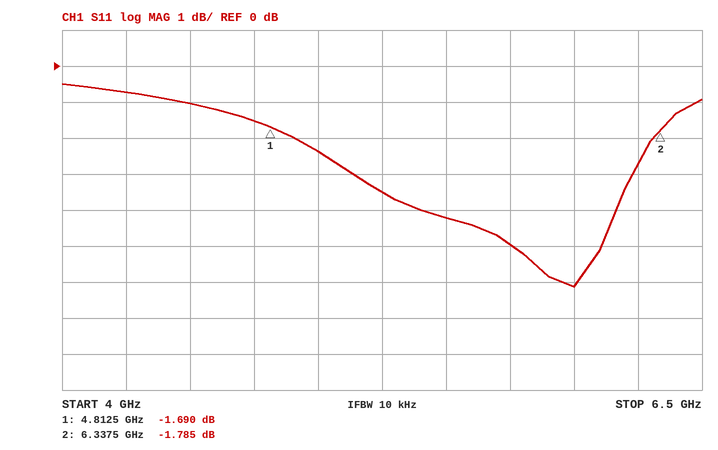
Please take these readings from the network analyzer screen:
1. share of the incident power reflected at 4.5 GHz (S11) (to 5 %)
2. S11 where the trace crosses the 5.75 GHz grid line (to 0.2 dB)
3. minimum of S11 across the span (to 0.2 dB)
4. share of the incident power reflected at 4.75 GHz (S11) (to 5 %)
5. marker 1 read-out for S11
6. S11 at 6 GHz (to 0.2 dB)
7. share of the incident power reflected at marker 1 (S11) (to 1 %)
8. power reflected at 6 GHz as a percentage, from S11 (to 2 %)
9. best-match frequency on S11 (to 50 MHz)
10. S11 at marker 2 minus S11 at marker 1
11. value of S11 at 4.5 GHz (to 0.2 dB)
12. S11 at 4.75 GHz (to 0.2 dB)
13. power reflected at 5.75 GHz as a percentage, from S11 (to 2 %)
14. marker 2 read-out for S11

80 %
-5.0 dB
-6.2 dB
70 %
-1.690 dB
-6.2 dB
68 %
24 %
6.00 GHz
-0.095 dB
-1.0 dB
-1.6 dB
32 %
-1.785 dB
